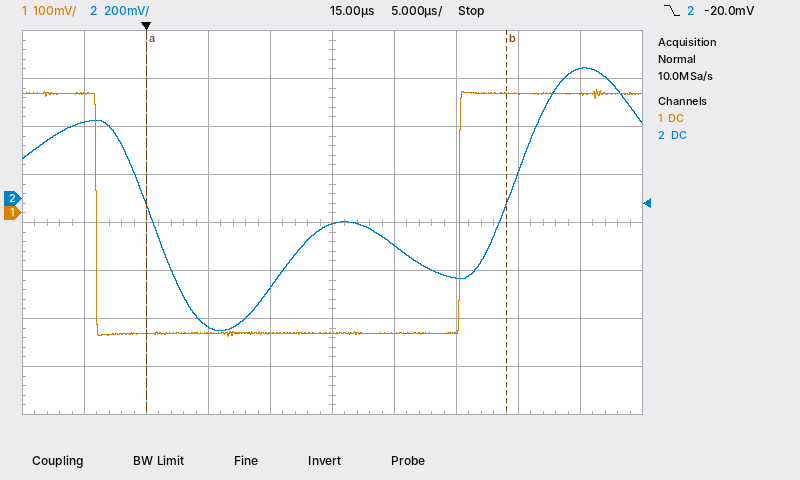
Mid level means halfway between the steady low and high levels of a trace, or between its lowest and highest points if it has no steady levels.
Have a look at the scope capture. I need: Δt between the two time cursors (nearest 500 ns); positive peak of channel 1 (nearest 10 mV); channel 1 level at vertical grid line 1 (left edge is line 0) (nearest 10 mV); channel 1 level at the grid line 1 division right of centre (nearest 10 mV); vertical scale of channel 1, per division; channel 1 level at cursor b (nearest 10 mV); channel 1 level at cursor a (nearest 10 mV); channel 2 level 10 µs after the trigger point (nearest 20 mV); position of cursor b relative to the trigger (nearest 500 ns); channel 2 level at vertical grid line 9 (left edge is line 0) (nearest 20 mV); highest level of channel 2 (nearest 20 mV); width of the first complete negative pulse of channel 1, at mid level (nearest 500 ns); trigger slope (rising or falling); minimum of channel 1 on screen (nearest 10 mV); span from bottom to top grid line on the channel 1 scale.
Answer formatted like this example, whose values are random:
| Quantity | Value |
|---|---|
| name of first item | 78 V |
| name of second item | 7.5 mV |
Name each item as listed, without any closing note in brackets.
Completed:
| Quantity | Value |
|---|---|
| Δt between the two time cursors | 29.0 µs |
| positive peak of channel 1 | 260 mV |
| channel 1 level at vertical grid line 1 (left edge is line 0) | 250 mV |
| channel 1 level at the grid line 1 division right of centre | -250 mV |
| vertical scale of channel 1, per division | 100 mV |
| channel 1 level at cursor b | 250 mV |
| channel 1 level at cursor a | -250 mV |
| channel 2 level 10 µs after the trigger point | -380 mV |
| position of cursor b relative to the trigger | +29.0 µs |
| channel 2 level at vertical grid line 9 (left edge is line 0) | 540 mV |
| highest level of channel 2 | 540 mV |
| width of the first complete negative pulse of channel 1, at mid level | 29.5 µs |
| trigger slope | falling |
| minimum of channel 1 on screen | -260 mV |
| span from bottom to top grid line on the channel 1 scale | 800 mV |
